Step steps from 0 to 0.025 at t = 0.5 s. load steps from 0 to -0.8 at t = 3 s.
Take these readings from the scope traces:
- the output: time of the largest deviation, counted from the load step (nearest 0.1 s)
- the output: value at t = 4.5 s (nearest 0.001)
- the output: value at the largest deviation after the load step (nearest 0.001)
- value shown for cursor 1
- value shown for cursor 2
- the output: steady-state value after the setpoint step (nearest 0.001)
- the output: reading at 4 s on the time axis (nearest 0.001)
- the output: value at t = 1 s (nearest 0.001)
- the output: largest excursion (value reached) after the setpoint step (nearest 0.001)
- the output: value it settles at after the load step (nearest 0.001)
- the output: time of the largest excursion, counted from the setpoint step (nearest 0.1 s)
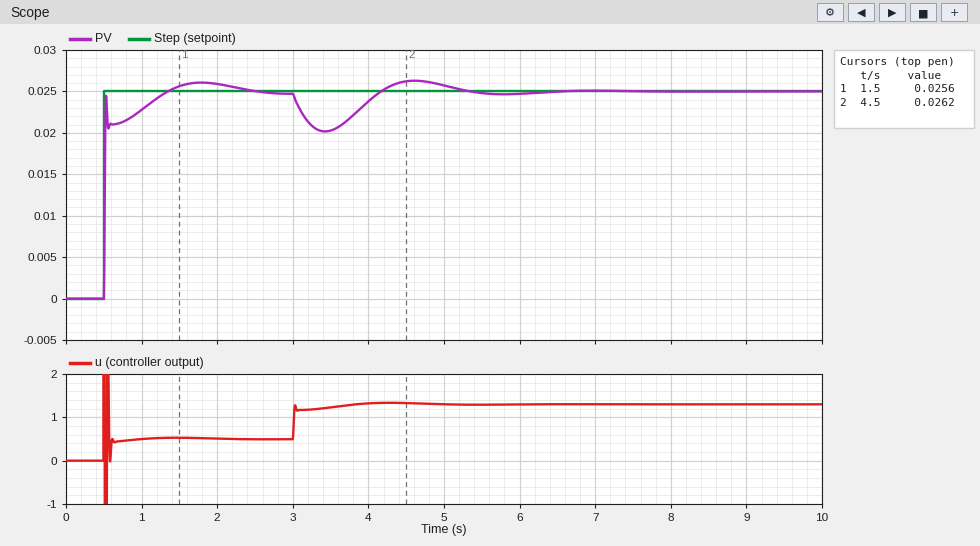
0.4 s
0.026
0.020
0.0256
0.0262
0.025
0.024
0.023
0.026
0.025
1.3 s
